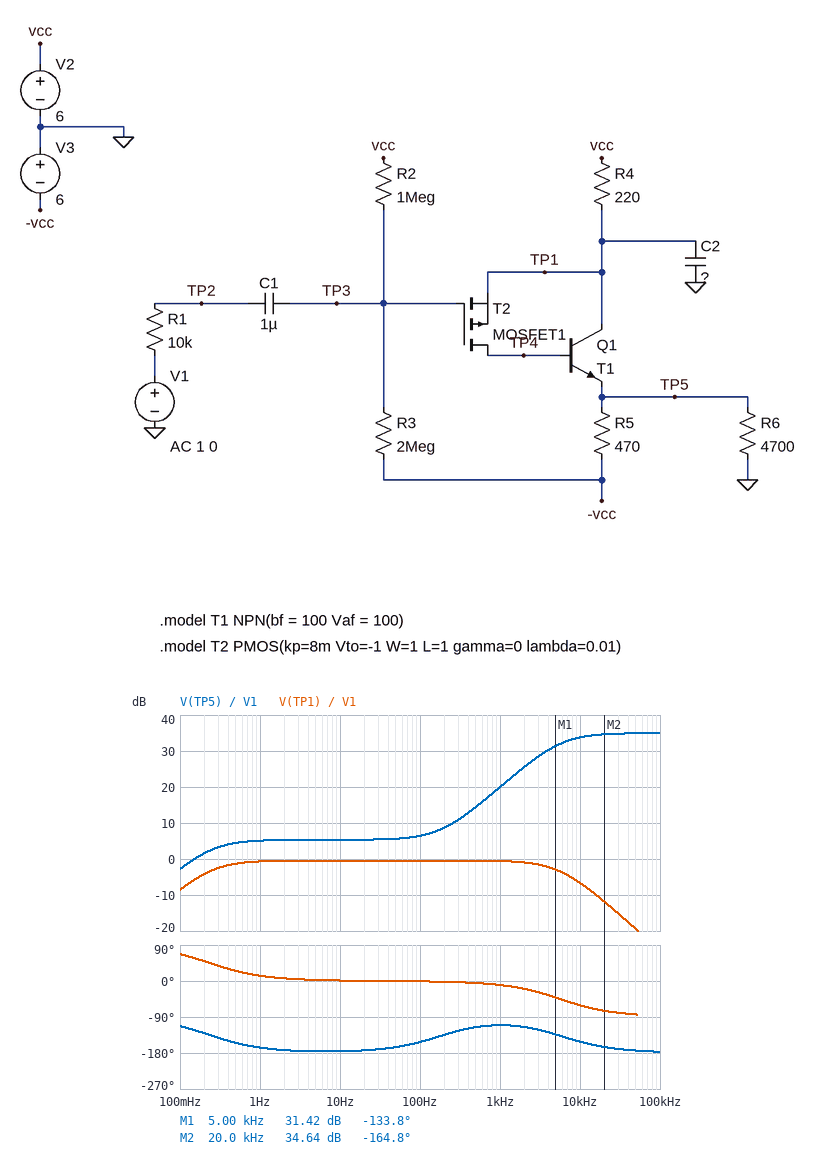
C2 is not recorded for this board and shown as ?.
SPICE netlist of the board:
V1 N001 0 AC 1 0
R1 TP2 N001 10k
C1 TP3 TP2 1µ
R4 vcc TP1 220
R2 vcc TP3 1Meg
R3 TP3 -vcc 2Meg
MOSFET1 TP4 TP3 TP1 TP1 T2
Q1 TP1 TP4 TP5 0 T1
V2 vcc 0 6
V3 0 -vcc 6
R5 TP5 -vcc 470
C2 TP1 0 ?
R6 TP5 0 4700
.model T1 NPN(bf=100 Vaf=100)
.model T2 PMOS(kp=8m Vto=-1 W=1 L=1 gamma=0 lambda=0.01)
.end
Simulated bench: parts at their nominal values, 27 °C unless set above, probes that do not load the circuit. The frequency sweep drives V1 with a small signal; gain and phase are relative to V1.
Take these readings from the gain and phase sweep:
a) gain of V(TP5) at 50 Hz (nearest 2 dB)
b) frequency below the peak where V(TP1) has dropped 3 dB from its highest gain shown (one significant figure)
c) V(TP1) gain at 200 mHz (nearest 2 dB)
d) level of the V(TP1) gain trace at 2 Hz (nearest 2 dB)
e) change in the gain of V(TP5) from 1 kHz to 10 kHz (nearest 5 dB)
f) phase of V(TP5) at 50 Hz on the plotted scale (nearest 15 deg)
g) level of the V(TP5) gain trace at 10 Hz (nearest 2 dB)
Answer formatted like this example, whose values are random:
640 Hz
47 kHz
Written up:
6 dB
200 mHz
-4 dB
0 dB
15 dB
-165 deg
6 dB
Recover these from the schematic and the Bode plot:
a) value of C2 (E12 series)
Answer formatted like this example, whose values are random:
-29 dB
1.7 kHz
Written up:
3.9 µF
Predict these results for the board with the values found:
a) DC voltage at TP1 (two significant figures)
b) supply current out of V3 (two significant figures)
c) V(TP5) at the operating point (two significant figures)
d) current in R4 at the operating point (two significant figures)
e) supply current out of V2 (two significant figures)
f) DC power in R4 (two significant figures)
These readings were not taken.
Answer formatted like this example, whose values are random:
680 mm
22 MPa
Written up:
3.2 V
13 mA
33 mV
13 mA
13 mA
36 mW
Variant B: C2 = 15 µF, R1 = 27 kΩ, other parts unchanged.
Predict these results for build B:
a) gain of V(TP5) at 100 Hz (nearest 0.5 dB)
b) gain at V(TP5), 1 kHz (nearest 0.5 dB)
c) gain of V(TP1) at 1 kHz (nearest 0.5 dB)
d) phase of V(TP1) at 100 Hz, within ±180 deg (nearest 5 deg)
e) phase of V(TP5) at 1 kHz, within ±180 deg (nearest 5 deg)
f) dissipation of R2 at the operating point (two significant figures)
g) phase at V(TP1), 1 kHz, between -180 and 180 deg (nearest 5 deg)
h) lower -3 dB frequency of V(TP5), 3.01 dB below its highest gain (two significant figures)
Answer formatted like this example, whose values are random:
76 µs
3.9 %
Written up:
12.5 dB
30.0 dB
-2.5 dB
-5 deg
-125 deg
16 µW
-35 deg
1.5 kHz
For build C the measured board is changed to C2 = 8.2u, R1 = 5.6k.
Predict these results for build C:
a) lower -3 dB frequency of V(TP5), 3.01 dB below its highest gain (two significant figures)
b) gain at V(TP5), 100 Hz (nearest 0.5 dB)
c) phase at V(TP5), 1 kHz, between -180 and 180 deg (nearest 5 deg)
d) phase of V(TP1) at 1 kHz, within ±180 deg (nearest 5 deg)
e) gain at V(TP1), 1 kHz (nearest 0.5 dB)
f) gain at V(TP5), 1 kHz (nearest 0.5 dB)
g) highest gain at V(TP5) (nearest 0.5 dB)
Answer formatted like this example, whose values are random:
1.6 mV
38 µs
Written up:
2.7 kHz
9.0 dB
-115 deg
-20 deg
-1.0 dB
26.0 dB
35.0 dB
